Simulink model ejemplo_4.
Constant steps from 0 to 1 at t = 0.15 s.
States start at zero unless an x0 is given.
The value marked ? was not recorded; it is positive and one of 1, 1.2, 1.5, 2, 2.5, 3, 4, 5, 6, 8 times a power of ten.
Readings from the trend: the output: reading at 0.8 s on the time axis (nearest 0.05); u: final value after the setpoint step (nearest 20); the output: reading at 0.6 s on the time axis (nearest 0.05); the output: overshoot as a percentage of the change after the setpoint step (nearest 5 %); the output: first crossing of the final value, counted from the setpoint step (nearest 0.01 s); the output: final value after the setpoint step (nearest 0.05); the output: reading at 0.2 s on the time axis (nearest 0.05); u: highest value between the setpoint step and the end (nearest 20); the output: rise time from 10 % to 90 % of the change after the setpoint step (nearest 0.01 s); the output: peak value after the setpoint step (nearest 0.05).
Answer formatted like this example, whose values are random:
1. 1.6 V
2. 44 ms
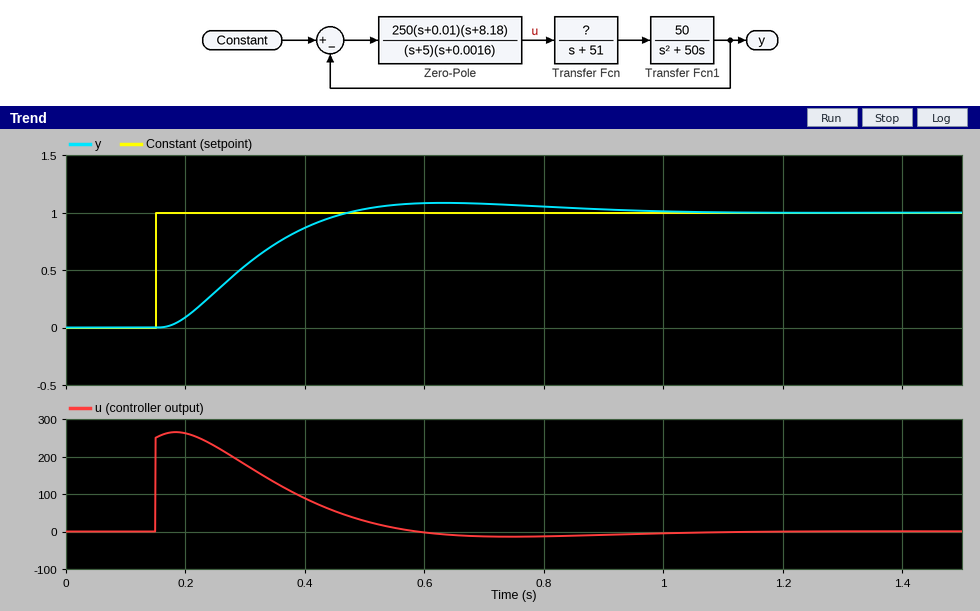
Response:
1. 1.05
2. 0
3. 1.10
4. 10 %
5. 0.32 s
6. 1.00
7. 0.10
8. 260
9. 0.21 s
10. 1.10
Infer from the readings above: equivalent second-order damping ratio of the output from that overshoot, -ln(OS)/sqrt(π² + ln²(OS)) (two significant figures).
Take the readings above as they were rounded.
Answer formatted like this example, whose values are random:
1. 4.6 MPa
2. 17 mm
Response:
1. 0.59
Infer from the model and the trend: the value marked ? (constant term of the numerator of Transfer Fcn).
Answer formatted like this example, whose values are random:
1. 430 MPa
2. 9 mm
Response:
1. 1
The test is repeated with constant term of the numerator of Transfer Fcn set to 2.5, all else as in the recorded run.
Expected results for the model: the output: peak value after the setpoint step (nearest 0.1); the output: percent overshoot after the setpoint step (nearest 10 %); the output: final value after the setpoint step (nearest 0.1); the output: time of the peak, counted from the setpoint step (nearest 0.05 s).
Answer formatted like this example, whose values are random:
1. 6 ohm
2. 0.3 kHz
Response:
1. 1.2
2. 20 %
3. 1.0
4. 0.20 s
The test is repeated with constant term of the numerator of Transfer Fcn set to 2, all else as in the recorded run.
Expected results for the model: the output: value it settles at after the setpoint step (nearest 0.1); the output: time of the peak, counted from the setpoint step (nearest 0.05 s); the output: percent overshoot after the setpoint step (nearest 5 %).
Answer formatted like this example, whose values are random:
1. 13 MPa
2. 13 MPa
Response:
1. 1.0
2. 0.25 s
3. 15 %
